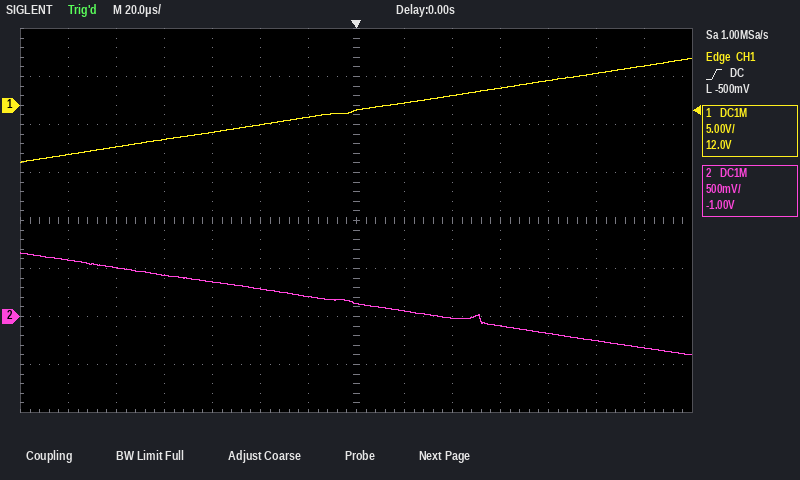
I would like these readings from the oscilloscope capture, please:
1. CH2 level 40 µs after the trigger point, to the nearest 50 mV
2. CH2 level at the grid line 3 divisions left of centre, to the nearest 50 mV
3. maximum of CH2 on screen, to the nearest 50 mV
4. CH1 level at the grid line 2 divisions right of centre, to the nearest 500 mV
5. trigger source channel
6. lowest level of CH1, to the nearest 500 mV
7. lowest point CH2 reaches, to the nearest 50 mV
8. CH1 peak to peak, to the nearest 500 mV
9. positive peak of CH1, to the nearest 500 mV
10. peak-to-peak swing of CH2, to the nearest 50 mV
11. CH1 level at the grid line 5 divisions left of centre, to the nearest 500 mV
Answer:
0 mV
350 mV
650 mV
1.0 V
CH1
-6.0 V
-400 mV
11.0 V
5.0 V
1.05 V
-4.5 V
